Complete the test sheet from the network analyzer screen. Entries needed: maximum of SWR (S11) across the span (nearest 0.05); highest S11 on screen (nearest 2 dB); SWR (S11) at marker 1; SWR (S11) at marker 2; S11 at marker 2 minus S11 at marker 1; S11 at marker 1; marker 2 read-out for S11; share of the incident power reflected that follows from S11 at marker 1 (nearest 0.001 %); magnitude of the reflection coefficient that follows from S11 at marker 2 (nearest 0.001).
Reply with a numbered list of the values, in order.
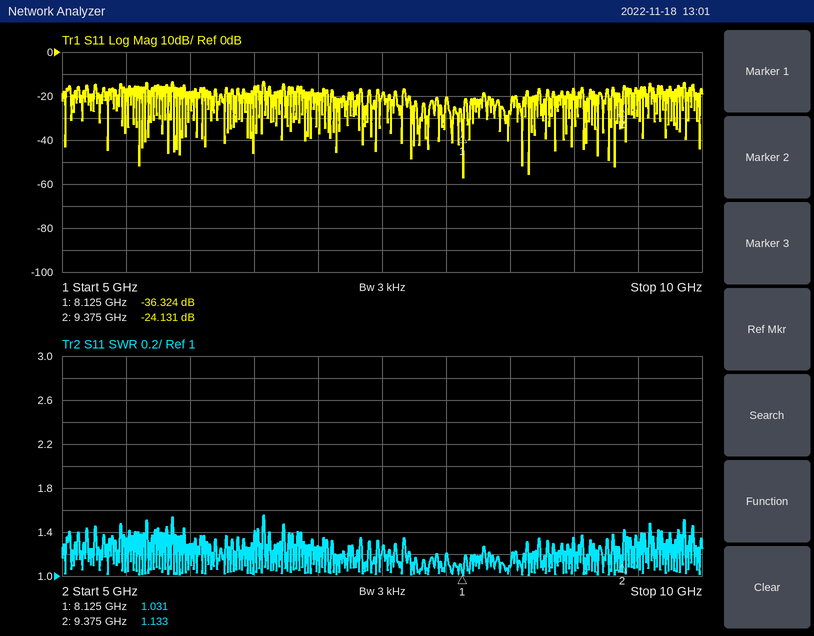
1. 1.55
2. -14 dB
3. 1.031
4. 1.133
5. 12.193 dB
6. -36.324 dB
7. -24.131 dB
8. 0.023 %
9. 0.062
